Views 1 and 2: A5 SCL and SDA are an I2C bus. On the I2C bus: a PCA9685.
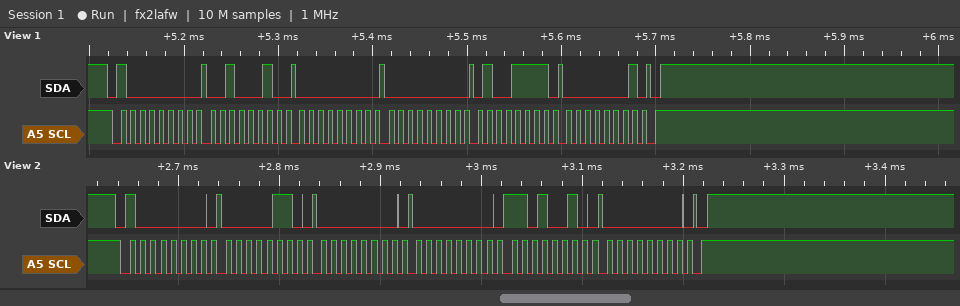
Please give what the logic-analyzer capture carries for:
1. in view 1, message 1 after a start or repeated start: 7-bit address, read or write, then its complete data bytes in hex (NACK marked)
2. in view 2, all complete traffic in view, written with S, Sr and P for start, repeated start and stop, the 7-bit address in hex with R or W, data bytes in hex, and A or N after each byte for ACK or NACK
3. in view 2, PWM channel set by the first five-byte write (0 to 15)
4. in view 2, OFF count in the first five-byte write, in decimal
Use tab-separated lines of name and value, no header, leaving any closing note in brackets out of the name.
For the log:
in view 1, message 1 after a start or repeated start: 7-bit address, read or write, then its complete data bytes in hex	0x40 write: 22 00 00 4F 01
in view 2, all complete traffic in view, written with S, Sr and P for start, repeated start and stop, the 7-bit address in hex with R or W, data bytes in hex, and A or N after each byte for ACK or NACK	S 40W A 06 A 00 A 00 A D2 A 00 A P
in view 2, PWM channel set by the first five-byte write	0
in view 2, OFF count in the first five-byte write, in decimal	210
